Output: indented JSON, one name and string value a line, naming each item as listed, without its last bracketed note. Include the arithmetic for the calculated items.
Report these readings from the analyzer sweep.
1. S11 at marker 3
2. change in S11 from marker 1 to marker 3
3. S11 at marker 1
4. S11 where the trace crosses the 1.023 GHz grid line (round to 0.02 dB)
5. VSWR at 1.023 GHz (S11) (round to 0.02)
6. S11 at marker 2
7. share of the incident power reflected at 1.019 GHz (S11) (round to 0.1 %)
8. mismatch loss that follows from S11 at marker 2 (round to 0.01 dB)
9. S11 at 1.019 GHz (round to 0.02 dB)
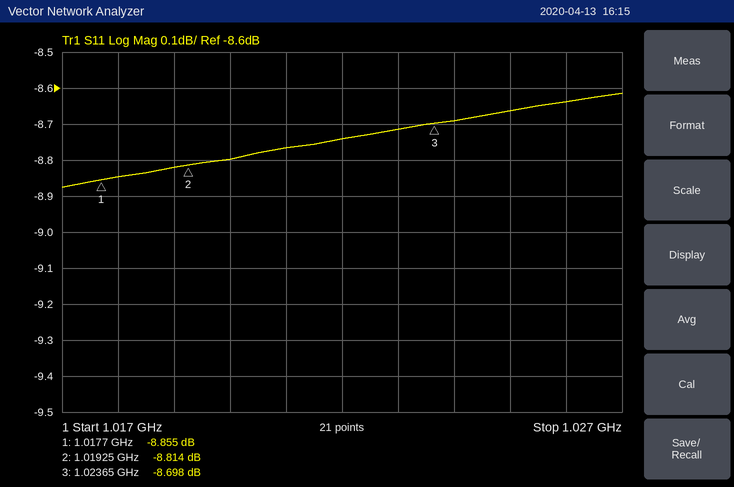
{
  "S11 at marker 3": "-8.698 dB",
  "change in S11 from marker 1 to marker 3": "-8.698 − (-8.855) = 0.157 dB",
  "S11 at marker 1": "-8.855 dB",
  "S11 where the trace crosses the 1.023 GHz grid line": "-8.72 dB",
  "VSWR at 1.023 GHz (S11)": "|Γ| = 10^(-8.72/20) = 0.3664; VSWR = (1 + 0.3664)/(1 − 0.3664) ≈ 2.16",
  "S11 at marker 2": "-8.814 dB",
  "share of the incident power reflected at 1.019 GHz (S11)": "10^(-8.82/10) ≈ 13.1 %",
  "mismatch loss that follows from S11 at marker 2": "−10 log10(1 − 10^(-8.814/10)) ≈ 0.61 dB",
  "S11 at 1.019 GHz": "-8.82 dB"
}
